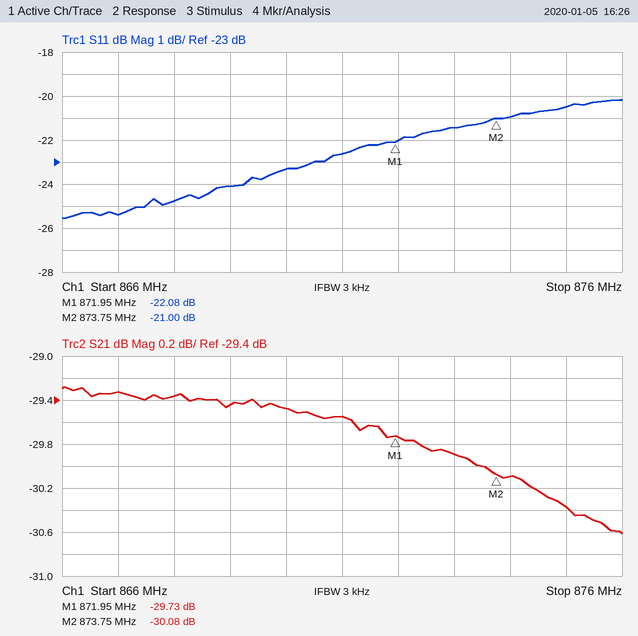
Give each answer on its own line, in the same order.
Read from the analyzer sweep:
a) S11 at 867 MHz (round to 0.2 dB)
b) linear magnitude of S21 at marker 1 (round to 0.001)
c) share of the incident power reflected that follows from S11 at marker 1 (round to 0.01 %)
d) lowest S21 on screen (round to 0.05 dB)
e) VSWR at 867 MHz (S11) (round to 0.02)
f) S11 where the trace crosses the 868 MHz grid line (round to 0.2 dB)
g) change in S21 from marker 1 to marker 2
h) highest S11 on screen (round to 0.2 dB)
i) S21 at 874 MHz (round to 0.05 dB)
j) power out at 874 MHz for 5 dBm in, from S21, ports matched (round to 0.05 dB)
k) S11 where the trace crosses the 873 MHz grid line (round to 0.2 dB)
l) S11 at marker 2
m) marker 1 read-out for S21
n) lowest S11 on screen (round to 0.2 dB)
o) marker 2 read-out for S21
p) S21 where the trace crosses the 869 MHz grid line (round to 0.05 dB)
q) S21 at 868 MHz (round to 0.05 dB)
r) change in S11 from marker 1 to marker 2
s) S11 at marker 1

-25.4 dB
0.033
0.62 %
-30.60 dB
1.12
-24.8 dB
-0.35 dB
-20.2 dB
-30.10 dB
-25.10 dBm
-21.4 dB
-21.00 dB
-29.73 dB
-25.6 dB
-30.08 dB
-29.45 dB
-29.35 dB
1.08 dB
-22.08 dB
